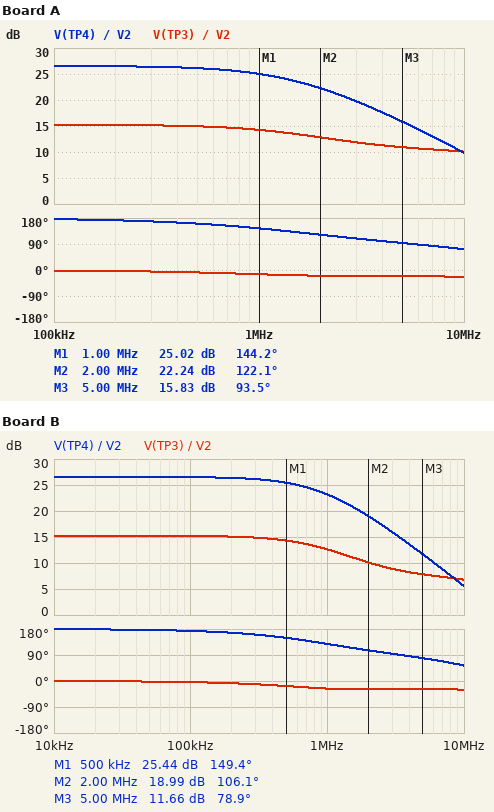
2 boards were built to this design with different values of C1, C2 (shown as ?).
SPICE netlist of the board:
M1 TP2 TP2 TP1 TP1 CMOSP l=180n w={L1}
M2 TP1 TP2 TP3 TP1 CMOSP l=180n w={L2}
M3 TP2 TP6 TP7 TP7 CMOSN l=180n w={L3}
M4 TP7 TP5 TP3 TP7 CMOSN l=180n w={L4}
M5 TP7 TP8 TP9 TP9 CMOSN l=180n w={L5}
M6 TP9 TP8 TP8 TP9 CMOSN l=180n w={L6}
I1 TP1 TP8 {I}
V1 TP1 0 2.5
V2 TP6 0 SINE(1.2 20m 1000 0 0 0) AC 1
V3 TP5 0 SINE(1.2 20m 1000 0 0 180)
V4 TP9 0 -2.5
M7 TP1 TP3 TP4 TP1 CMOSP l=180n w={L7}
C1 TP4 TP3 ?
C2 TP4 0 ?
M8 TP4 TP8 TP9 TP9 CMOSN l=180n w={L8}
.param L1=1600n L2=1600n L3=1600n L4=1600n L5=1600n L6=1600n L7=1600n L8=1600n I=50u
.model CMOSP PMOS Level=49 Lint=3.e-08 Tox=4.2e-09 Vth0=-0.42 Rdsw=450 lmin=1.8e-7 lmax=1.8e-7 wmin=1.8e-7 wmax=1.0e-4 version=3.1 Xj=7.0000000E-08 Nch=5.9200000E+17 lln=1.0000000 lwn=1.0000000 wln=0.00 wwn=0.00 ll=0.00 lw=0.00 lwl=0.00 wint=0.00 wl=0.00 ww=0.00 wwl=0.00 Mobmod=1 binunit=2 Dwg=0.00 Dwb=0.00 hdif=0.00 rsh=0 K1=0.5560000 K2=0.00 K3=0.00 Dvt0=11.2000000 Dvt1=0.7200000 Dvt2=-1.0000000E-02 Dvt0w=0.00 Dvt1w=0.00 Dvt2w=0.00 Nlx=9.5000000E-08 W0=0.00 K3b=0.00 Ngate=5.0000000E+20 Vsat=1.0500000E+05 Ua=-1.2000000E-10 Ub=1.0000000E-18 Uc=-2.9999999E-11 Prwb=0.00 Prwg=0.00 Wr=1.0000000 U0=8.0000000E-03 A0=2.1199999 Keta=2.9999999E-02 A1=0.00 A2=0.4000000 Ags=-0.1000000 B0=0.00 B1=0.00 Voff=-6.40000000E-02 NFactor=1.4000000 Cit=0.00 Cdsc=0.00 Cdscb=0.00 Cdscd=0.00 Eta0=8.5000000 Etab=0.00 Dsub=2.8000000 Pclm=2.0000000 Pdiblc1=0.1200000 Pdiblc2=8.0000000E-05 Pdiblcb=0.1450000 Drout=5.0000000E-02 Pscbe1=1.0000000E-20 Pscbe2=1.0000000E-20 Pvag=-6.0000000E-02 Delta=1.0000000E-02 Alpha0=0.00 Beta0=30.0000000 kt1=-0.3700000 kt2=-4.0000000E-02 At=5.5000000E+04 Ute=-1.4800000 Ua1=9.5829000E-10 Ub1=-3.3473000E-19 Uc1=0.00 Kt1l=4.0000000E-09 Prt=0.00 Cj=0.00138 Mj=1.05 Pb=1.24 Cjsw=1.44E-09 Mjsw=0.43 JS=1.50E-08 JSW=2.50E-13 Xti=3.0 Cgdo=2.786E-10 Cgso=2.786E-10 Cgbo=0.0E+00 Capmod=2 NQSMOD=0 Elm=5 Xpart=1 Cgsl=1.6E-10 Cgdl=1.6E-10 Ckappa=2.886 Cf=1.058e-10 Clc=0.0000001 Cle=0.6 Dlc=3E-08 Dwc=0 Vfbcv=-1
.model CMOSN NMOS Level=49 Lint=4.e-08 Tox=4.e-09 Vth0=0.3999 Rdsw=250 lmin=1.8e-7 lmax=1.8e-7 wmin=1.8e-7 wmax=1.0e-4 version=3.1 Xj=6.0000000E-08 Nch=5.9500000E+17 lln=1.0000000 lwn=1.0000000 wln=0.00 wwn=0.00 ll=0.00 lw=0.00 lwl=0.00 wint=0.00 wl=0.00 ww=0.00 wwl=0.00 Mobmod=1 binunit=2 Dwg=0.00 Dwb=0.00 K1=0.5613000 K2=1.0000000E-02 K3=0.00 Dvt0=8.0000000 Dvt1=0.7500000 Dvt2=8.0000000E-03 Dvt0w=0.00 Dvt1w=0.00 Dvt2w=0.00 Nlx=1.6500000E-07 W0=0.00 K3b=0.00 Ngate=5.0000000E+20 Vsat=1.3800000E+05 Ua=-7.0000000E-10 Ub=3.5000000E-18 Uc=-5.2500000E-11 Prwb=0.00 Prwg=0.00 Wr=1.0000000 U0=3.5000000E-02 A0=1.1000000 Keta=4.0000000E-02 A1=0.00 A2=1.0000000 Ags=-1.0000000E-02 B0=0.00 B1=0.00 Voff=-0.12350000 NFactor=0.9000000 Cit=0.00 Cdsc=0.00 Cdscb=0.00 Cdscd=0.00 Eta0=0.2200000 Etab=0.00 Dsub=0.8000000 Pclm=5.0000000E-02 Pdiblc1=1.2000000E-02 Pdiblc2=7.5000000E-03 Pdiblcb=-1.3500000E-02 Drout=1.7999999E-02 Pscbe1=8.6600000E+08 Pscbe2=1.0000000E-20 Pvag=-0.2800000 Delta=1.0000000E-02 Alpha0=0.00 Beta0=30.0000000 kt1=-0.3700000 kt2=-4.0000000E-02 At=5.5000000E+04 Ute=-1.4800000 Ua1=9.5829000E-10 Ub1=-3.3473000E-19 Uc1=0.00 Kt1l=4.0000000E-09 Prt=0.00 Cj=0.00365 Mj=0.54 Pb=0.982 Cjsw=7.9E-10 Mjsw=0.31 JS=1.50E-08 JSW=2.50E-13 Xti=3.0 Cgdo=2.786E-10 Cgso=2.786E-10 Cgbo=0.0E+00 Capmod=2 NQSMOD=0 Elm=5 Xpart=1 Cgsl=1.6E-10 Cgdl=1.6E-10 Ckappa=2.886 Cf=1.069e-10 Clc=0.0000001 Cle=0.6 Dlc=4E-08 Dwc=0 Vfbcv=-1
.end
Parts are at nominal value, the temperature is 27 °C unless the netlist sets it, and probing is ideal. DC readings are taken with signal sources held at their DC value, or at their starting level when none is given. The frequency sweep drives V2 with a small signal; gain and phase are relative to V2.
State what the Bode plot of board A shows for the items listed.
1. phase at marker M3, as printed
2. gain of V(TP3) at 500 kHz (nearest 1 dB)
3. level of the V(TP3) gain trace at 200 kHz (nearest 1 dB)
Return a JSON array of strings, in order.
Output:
["93.5 deg", "15 dB", "15 dB"]
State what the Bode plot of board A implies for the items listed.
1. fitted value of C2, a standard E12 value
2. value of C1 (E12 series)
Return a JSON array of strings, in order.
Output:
["5.6 pF", "1 pF"]
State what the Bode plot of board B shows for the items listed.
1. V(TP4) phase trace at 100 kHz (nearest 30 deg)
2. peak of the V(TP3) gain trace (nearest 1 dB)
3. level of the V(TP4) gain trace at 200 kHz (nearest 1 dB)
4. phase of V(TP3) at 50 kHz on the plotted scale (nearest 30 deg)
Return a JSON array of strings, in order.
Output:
["180 deg", "15 dB", "26 dB", "0 deg"]
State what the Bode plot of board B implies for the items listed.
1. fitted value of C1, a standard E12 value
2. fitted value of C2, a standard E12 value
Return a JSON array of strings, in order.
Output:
["2.2 pF", "5.6 pF"]
